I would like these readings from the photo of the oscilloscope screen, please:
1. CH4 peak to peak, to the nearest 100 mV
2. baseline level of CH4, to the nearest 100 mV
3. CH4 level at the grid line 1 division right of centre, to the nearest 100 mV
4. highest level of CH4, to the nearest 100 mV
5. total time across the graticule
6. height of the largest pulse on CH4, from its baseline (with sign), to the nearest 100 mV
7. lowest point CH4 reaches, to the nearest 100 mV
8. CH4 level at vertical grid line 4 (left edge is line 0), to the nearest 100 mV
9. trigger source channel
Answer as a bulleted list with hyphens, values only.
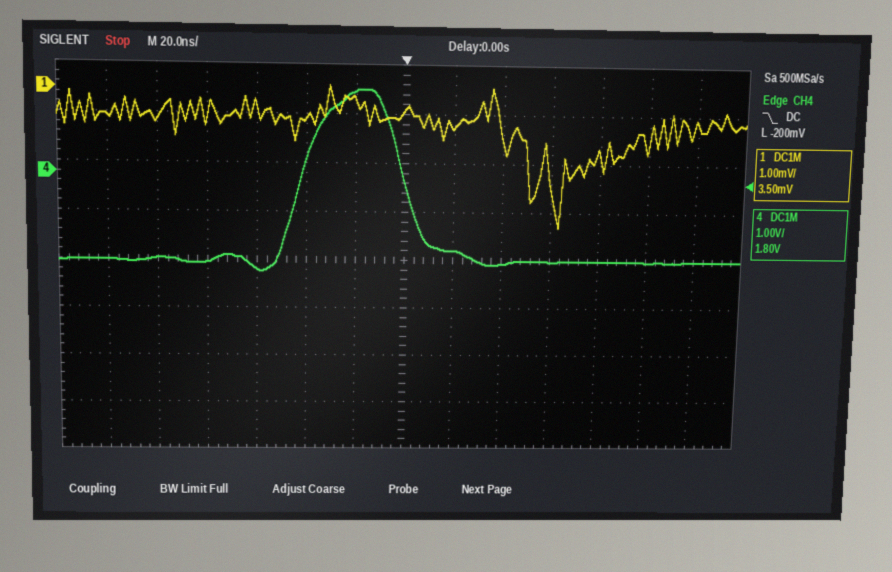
- 3.7 V
- -1.8 V
- -1.6 V
- 1.7 V
- 280 ns
- +3.5 V
- -2.0 V
- -2.0 V
- CH4
